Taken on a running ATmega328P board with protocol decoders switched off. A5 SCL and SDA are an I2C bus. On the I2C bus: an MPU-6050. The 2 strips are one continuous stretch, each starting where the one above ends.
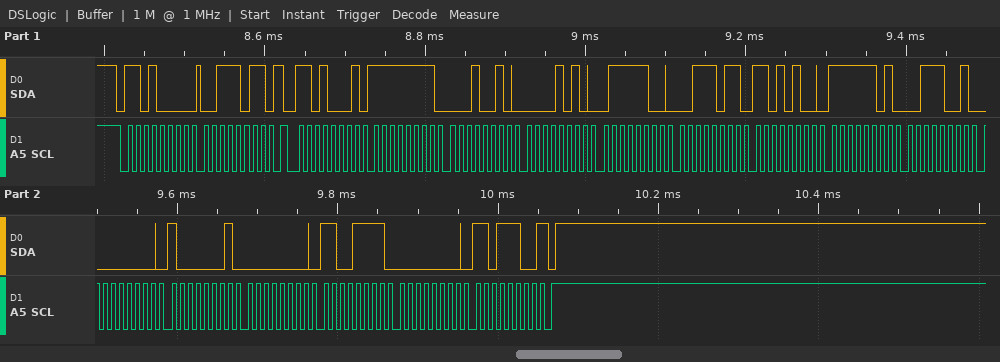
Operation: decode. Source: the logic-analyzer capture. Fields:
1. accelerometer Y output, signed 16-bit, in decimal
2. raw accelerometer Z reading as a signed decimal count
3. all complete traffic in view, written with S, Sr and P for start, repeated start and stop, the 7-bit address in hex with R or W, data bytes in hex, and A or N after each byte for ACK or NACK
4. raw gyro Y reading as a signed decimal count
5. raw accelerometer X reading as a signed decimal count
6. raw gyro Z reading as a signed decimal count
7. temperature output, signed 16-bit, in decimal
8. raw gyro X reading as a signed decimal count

2684
15316
S 68W A 3B A Sr 68R A FF A 12 A 0A A 7C A 3B A D4 A FD A 39 A 00 A 81 A 00 A CF A 00 A DC N P
207
-238
220
-711
129
